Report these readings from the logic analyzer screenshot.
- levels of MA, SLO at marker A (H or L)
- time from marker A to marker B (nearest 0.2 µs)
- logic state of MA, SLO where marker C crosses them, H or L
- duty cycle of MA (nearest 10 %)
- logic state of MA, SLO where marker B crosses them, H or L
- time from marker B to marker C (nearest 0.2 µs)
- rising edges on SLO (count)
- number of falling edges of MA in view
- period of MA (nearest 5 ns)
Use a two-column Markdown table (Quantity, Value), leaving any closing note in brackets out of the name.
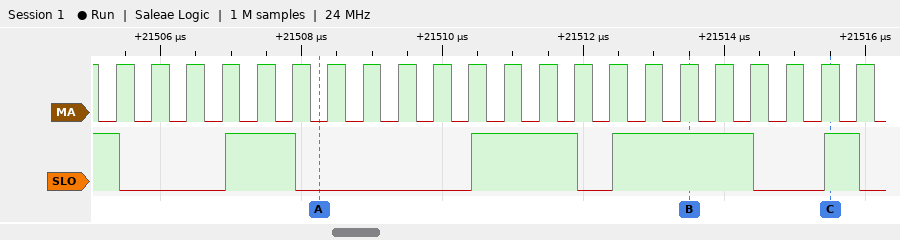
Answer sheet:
| Quantity | Value |
|---|---|
| levels of MA, SLO at marker A | MA=L, SLO=L |
| time from marker A to marker B | 5.2 µs |
| logic state of MA, SLO where marker C crosses them, H or L | MA=H, SLO=H |
| duty cycle of MA | 50 % |
| logic state of MA, SLO where marker B crosses them, H or L | MA=H, SLO=H |
| time from marker B to marker C | 2 µs |
| rising edges on SLO | 4 |
| number of falling edges of MA in view | 23 |
| period of MA | 500 ns |
